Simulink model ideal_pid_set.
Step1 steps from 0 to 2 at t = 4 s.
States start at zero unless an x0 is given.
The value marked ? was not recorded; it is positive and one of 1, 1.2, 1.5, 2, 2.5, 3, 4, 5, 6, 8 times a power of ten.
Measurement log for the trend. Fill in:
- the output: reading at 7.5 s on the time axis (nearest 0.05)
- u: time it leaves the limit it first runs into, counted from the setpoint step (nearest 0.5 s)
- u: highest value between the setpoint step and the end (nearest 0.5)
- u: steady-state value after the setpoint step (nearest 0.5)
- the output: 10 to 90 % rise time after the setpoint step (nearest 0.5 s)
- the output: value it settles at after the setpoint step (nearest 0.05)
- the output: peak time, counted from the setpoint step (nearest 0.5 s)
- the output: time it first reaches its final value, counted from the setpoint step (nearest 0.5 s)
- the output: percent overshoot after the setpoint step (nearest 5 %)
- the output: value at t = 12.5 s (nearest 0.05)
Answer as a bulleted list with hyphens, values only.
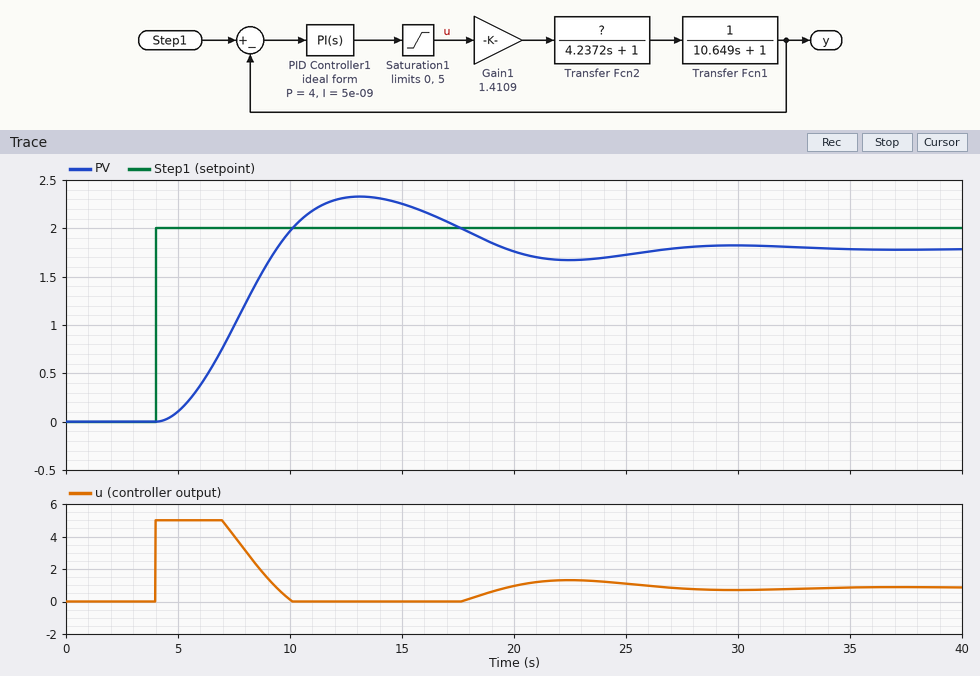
- 1.00
- 3.0 s
- 5.0
- 1.0
- 3.5 s
- 1.80
- 9.0 s
- 5.5 s
- 30 %
- 2.30
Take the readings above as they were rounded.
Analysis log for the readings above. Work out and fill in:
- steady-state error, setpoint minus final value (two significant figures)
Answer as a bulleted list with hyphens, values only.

- 0.20
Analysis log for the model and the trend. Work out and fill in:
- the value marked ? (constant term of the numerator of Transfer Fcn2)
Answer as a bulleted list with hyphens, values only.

- 1.5
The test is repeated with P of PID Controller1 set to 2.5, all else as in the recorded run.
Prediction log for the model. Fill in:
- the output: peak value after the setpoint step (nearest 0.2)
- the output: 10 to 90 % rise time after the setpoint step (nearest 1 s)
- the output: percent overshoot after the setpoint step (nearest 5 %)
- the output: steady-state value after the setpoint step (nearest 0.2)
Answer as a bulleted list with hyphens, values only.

- 2.0
- 4 s
- 20 %
- 1.6
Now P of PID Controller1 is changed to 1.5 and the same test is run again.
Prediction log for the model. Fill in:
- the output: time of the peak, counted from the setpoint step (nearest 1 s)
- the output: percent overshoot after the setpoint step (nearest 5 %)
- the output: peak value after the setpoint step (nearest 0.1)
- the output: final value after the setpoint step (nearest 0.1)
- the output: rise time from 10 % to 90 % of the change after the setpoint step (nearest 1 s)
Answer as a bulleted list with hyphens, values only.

- 12 s
- 15 %
- 1.7
- 1.5
- 6 s
